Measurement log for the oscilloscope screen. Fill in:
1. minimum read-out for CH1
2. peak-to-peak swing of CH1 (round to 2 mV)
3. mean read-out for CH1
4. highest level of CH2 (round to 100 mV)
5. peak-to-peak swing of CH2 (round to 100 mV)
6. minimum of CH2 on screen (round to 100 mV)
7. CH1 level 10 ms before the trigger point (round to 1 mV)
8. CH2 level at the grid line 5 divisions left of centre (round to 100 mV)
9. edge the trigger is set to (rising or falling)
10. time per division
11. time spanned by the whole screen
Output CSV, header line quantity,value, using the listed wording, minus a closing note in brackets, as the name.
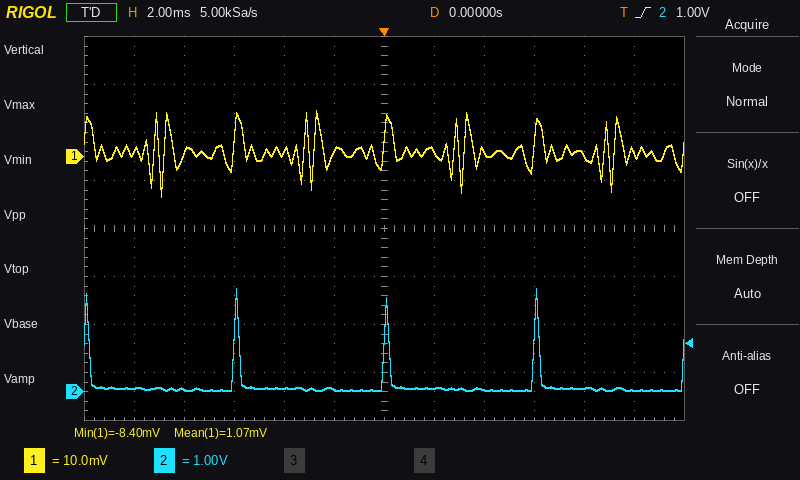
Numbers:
quantity,value
minimum read-out for CH1,-8.40 mV
peak-to-peak swing of CH1,18 mV
mean read-out for CH1,1.07 mV
highest level of CH2,2.1 V
peak-to-peak swing of CH2,2.1 V
minimum of CH2 on screen,0.0 V
CH1 level 10 ms before the trigger point,1 mV
CH2 level at the grid line 5 divisions left of centre,100 mV
edge the trigger is set to,rising
time per division,2 ms
time spanned by the whole screen,24 ms
